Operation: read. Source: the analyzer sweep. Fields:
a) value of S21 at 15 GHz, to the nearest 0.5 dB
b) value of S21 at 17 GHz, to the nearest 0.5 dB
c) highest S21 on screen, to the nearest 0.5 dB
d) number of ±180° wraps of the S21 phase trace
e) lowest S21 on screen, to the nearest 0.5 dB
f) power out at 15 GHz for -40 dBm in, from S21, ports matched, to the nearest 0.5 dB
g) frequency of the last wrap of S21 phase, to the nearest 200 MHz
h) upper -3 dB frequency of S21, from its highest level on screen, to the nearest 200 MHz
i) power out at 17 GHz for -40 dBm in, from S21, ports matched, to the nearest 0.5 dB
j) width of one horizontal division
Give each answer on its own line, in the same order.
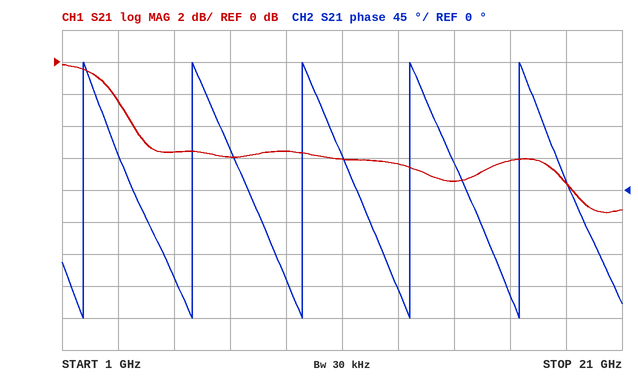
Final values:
-7.5 dB
-6.0 dB
0.0 dB
5
-9.5 dB
-47.5 dBm
17.4 GHz
3.2 GHz
-46.0 dBm
2 GHz
